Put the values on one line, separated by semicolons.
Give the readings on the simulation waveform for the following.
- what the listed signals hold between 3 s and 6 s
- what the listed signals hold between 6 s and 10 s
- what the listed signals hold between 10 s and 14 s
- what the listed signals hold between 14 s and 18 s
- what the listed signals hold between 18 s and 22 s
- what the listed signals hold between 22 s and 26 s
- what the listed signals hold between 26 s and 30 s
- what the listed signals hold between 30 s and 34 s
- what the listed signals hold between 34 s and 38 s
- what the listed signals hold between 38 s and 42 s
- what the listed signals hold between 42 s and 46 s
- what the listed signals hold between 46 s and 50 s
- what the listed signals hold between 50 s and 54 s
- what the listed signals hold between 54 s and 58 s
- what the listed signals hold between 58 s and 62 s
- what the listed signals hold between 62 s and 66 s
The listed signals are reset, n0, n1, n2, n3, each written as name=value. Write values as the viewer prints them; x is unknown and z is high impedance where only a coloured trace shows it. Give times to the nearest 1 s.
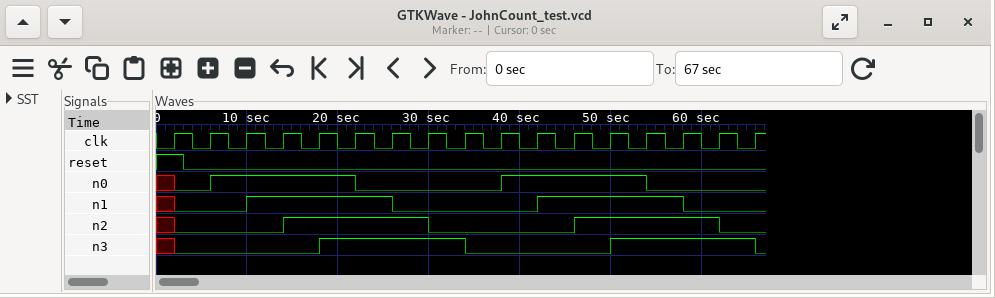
reset=0, n0=0, n1=0, n2=0, n3=0; reset=0, n0=1, n1=0, n2=0, n3=0; reset=0, n0=1, n1=1, n2=0, n3=0; reset=0, n0=1, n1=1, n2=1, n3=0; reset=0, n0=1, n1=1, n2=1, n3=1; reset=0, n0=0, n1=1, n2=1, n3=1; reset=0, n0=0, n1=0, n2=1, n3=1; reset=0, n0=0, n1=0, n2=0, n3=1; reset=0, n0=0, n1=0, n2=0, n3=0; reset=0, n0=1, n1=0, n2=0, n3=0; reset=0, n0=1, n1=1, n2=0, n3=0; reset=0, n0=1, n1=1, n2=1, n3=0; reset=0, n0=1, n1=1, n2=1, n3=1; reset=0, n0=0, n1=1, n2=1, n3=1; reset=0, n0=0, n1=0, n2=1, n3=1; reset=0, n0=0, n1=0, n2=0, n3=1
